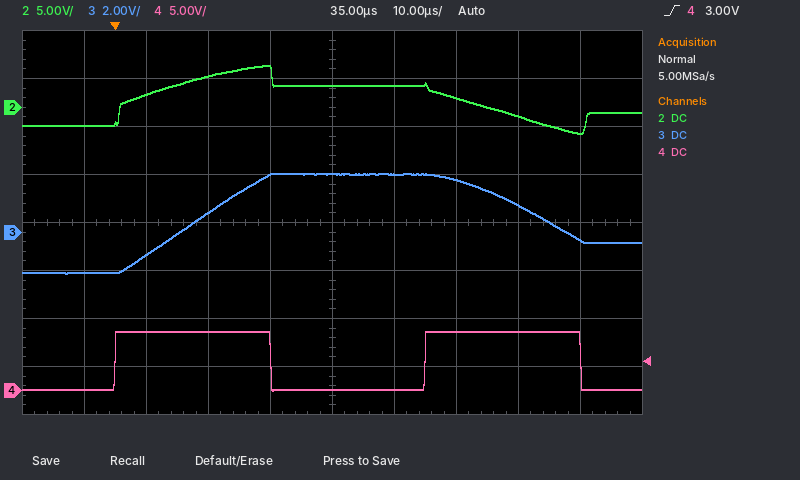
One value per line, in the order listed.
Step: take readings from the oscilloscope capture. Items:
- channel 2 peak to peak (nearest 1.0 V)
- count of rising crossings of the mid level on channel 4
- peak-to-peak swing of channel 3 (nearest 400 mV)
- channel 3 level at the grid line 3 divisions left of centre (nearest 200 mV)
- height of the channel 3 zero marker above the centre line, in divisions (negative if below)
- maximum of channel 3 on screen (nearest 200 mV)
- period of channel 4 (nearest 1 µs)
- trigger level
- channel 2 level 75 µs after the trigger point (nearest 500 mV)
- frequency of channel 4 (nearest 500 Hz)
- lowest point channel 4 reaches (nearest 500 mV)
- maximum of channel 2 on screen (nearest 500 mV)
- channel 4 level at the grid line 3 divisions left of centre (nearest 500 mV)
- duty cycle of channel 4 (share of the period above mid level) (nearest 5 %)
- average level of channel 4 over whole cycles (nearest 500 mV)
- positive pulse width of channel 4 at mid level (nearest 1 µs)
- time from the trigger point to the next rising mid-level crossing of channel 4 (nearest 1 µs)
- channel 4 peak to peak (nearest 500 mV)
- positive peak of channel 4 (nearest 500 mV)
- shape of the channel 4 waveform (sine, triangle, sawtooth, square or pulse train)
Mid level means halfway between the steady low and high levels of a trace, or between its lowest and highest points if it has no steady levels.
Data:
7.0 V
2
4.0 V
-1.0 V
-0.2 div
2.4 V
50 µs
3.00 V
-2.5 V
20.0 kHz
0.0 V
4.5 V
6.0 V
50 %
3.0 V
25 µs
50 µs
6.0 V
6.0 V
square
